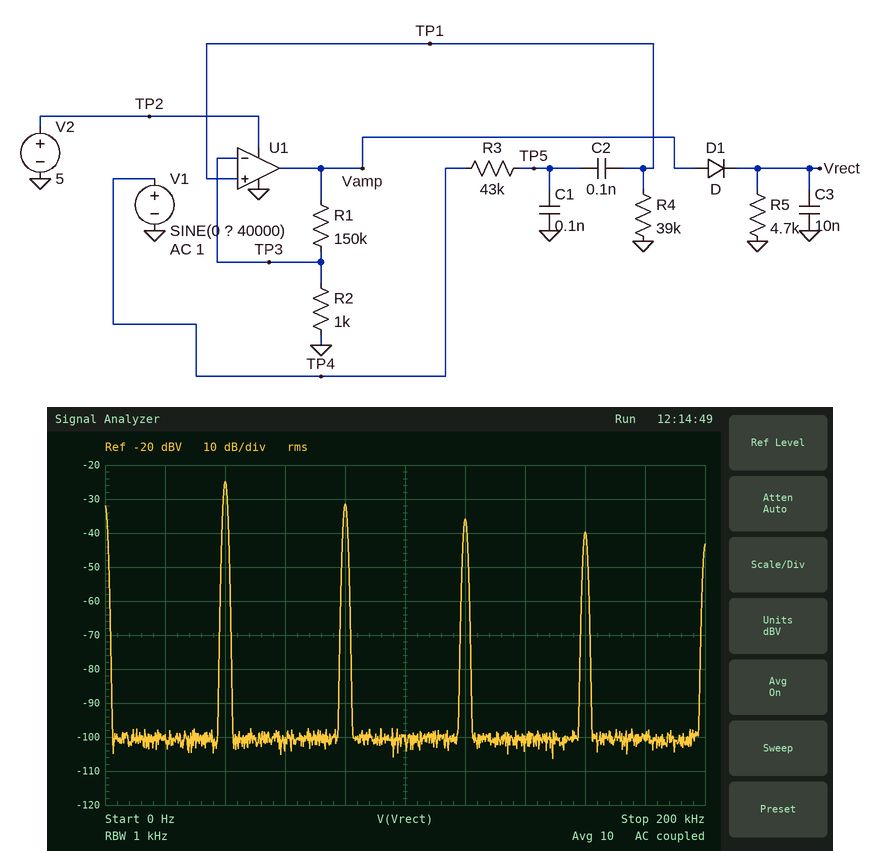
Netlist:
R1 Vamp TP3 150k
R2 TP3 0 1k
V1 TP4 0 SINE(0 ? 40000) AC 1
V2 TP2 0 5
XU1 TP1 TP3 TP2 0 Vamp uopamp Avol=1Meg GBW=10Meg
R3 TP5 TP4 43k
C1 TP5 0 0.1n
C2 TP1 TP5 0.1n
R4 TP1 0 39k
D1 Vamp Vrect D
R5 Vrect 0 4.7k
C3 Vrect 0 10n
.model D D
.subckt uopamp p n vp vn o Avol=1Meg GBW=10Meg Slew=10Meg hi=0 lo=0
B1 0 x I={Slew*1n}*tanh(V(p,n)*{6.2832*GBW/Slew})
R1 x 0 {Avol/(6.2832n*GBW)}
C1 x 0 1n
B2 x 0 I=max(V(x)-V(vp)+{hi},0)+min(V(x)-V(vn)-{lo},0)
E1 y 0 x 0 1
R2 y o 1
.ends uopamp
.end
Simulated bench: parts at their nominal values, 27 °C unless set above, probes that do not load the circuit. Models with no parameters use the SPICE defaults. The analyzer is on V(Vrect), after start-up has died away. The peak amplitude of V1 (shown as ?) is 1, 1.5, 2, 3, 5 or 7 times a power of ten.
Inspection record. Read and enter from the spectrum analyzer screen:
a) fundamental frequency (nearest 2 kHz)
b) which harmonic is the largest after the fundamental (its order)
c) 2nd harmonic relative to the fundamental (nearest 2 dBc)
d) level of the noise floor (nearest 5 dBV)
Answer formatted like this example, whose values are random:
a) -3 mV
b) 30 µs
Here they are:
a) 40 kHz
b) 2
c) -6 dBc
d) -100 dBV
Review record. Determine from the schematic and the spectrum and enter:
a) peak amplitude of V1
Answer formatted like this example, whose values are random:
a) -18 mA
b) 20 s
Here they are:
a) 30 mV
